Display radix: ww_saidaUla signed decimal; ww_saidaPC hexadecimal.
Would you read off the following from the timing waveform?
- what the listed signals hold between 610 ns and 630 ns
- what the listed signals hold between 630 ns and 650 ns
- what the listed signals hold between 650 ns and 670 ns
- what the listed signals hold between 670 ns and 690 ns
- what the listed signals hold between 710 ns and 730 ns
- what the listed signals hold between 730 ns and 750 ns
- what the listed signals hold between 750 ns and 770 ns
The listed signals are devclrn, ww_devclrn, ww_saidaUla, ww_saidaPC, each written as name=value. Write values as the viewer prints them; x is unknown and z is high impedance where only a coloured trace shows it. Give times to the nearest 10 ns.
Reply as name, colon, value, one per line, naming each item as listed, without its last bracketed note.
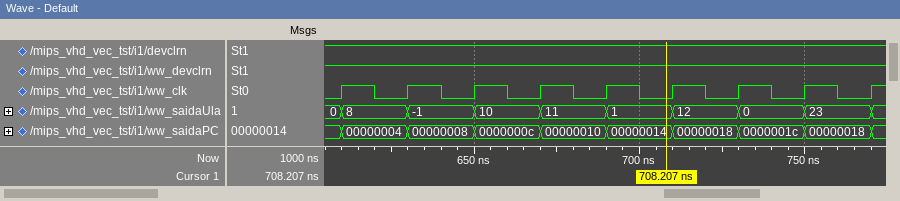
what the listed signals hold between 610 ns and 630 ns: devclrn=1, ww_devclrn=1, ww_saidaUla=8, ww_saidaPC=00000004
what the listed signals hold between 630 ns and 650 ns: devclrn=1, ww_devclrn=1, ww_saidaUla=-1, ww_saidaPC=00000008
what the listed signals hold between 650 ns and 670 ns: devclrn=1, ww_devclrn=1, ww_saidaUla=10, ww_saidaPC=0000000c
what the listed signals hold between 670 ns and 690 ns: devclrn=1, ww_devclrn=1, ww_saidaUla=11, ww_saidaPC=00000010
what the listed signals hold between 710 ns and 730 ns: devclrn=1, ww_devclrn=1, ww_saidaUla=12, ww_saidaPC=00000018
what the listed signals hold between 730 ns and 750 ns: devclrn=1, ww_devclrn=1, ww_saidaUla=0, ww_saidaPC=0000001c
what the listed signals hold between 750 ns and 770 ns: devclrn=1, ww_devclrn=1, ww_saidaUla=23, ww_saidaPC=00000018
